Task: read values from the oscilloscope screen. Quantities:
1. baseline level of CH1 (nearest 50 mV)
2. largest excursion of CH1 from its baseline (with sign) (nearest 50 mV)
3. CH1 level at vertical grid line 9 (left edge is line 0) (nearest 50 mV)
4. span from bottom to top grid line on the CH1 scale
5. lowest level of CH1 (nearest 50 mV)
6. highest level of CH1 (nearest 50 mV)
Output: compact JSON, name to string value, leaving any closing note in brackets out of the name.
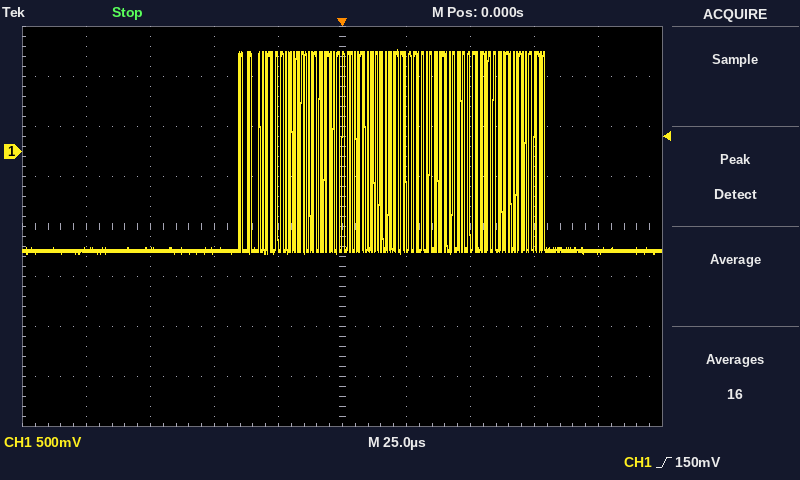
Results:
{"baseline level of CH1": "-1.00 V", "largest excursion of CH1 from its baseline (with sign)": "+2.00 V", "CH1 level at vertical grid line 9 (left edge is line 0)": "-1.00 V", "span from bottom to top grid line on the CH1 scale": "4 V", "lowest level of CH1": "-1.00 V", "highest level of CH1": "1.00 V"}
